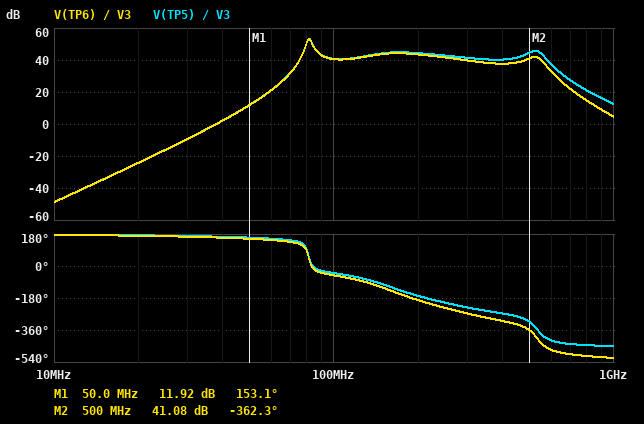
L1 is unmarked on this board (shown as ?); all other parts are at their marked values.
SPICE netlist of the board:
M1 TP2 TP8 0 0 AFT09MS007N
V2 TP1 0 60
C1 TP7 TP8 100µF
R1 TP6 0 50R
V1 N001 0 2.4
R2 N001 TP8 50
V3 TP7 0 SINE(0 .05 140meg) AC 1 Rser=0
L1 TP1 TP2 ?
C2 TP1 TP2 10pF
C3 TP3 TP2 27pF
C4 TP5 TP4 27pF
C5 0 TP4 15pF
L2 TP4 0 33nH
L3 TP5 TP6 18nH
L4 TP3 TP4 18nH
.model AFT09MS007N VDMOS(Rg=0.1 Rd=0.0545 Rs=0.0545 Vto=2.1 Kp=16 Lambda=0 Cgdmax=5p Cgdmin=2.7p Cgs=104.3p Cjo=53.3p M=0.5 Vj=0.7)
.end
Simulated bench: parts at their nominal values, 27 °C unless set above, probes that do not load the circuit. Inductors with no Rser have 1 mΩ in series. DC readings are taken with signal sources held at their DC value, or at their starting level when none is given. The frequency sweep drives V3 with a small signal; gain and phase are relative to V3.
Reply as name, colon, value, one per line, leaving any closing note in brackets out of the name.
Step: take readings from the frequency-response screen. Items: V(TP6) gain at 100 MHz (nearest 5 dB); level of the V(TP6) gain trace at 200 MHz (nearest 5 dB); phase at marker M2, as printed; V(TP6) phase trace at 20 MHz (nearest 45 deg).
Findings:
V(TP6) gain at 100 MHz: 40 dB
level of the V(TP6) gain trace at 200 MHz: 45 dB
phase at marker M2, as printed: -362.3 deg
V(TP6) phase trace at 20 MHz: 180 deg
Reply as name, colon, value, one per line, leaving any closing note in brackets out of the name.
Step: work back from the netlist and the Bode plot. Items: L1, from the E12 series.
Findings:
L1, from the E12 series: 56 nH
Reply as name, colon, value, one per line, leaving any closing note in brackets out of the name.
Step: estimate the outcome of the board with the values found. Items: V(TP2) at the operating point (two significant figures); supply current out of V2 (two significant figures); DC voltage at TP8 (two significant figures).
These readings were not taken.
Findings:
V(TP2) at the operating point: 60 V
supply current out of V2: 600 mA
DC voltage at TP8: 2.4 V
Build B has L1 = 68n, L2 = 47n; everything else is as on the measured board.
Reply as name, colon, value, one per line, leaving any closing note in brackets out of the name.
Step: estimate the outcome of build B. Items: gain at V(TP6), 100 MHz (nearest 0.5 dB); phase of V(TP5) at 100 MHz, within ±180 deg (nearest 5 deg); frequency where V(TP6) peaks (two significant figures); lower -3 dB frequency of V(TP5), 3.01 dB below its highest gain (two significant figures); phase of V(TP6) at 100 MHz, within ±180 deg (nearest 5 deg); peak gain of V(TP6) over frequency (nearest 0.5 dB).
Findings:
gain at V(TP6), 100 MHz: 42.5 dB
phase of V(TP5) at 100 MHz, within ±180 deg: -50 deg
frequency where V(TP6) peaks: 72 MHz
lower -3 dB frequency of V(TP5), 3.01 dB below its highest gain: 70 MHz
phase of V(TP6) at 100 MHz, within ±180 deg: -60 deg
peak gain of V(TP6) over frequency: 52.0 dB
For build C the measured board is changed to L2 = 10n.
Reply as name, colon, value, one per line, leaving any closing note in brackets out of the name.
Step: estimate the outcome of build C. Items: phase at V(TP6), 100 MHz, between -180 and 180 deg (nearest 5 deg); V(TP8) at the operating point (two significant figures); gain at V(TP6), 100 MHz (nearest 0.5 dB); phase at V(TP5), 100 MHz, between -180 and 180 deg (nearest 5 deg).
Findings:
phase at V(TP6), 100 MHz, between -180 and 180 deg: -50 deg
V(TP8) at the operating point: 2.4 V
gain at V(TP6), 100 MHz: 34.0 dB
phase at V(TP5), 100 MHz, between -180 and 180 deg: -35 deg
